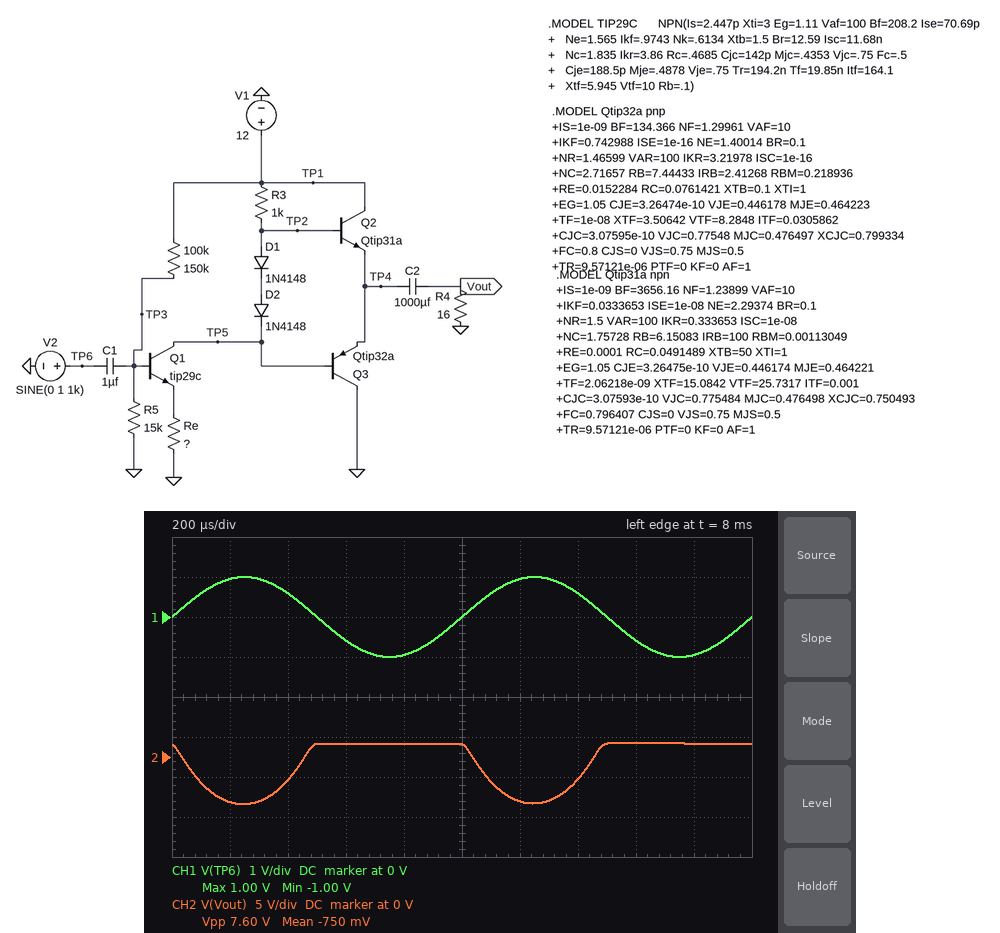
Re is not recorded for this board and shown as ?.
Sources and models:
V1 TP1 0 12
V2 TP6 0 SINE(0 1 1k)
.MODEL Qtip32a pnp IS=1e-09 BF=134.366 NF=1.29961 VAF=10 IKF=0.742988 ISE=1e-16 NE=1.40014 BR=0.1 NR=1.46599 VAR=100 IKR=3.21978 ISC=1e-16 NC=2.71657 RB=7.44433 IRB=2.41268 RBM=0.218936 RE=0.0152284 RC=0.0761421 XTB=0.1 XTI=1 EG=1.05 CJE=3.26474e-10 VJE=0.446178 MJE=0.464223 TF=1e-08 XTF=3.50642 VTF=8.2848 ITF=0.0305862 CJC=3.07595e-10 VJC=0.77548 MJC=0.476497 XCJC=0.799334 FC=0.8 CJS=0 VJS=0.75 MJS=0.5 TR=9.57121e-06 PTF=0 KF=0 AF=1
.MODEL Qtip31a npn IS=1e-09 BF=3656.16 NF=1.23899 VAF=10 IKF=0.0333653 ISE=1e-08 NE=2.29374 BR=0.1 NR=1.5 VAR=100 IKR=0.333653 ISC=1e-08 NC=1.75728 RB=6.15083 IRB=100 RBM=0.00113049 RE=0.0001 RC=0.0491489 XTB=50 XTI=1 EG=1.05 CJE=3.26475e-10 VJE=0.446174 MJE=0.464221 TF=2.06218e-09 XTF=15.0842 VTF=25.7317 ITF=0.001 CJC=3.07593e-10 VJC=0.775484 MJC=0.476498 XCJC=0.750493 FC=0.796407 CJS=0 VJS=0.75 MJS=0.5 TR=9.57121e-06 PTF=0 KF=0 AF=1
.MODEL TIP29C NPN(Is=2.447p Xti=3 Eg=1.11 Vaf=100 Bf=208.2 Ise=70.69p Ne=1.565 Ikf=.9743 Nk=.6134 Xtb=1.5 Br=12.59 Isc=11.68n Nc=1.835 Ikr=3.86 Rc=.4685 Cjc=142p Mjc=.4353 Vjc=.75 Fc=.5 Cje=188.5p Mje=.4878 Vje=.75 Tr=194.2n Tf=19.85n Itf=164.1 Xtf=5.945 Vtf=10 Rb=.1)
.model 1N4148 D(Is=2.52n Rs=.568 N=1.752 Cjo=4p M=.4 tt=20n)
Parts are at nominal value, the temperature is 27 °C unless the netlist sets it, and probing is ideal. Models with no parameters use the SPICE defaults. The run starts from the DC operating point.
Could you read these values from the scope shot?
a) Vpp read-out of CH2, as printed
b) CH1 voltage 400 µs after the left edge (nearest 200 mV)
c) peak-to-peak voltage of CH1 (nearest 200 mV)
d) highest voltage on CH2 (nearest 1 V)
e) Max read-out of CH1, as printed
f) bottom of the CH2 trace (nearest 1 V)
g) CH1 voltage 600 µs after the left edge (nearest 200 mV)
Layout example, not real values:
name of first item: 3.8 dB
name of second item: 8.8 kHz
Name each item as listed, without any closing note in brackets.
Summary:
Vpp read-out of CH2, as printed: 7.60 V
CH1 voltage 400 µs after the left edge: 600 mV
peak-to-peak voltage of CH1: 2.0 V
highest voltage on CH2: 2 V
Max read-out of CH1, as printed: 1.00 V
bottom of the CH2 trace: -6 V
CH1 voltage 600 µs after the left edge: -600 mV
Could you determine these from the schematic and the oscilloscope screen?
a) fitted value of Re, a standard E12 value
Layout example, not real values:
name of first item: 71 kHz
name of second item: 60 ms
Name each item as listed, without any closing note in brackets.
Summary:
fitted value of Re, a standard E12 value: 68 Ω
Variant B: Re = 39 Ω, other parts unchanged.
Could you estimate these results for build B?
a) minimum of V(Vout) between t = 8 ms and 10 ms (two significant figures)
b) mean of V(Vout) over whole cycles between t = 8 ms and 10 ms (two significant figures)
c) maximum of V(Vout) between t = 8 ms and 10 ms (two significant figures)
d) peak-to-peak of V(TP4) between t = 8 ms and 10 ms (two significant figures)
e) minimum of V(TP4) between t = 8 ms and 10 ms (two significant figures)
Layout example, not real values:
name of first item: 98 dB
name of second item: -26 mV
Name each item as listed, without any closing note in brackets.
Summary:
minimum of V(Vout) between t = 8 ms and 10 ms: -7.4 V
mean of V(Vout) over whole cycles between t = 8 ms and 10 ms: -850 mV
maximum of V(Vout) between t = 8 ms and 10 ms: 1.8 V
peak-to-peak of V(TP4) between t = 8 ms and 10 ms: 9.2 V
minimum of V(TP4) between t = 8 ms and 10 ms: 1.6 V
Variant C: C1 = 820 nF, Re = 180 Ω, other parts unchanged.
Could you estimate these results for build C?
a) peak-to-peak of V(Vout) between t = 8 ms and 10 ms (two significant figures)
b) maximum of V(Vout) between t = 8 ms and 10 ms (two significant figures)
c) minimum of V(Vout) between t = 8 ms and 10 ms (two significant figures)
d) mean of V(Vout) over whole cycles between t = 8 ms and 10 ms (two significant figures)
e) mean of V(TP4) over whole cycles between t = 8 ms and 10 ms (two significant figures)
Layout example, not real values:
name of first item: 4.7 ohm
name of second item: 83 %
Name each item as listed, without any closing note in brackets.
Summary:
peak-to-peak of V(Vout) between t = 8 ms and 10 ms: 4.2 V
maximum of V(Vout) between t = 8 ms and 10 ms: 1.1 V
minimum of V(Vout) between t = 8 ms and 10 ms: -3.1 V
mean of V(Vout) over whole cycles between t = 8 ms and 10 ms: -390 mV
mean of V(TP4) over whole cycles between t = 8 ms and 10 ms: 9.6 V
